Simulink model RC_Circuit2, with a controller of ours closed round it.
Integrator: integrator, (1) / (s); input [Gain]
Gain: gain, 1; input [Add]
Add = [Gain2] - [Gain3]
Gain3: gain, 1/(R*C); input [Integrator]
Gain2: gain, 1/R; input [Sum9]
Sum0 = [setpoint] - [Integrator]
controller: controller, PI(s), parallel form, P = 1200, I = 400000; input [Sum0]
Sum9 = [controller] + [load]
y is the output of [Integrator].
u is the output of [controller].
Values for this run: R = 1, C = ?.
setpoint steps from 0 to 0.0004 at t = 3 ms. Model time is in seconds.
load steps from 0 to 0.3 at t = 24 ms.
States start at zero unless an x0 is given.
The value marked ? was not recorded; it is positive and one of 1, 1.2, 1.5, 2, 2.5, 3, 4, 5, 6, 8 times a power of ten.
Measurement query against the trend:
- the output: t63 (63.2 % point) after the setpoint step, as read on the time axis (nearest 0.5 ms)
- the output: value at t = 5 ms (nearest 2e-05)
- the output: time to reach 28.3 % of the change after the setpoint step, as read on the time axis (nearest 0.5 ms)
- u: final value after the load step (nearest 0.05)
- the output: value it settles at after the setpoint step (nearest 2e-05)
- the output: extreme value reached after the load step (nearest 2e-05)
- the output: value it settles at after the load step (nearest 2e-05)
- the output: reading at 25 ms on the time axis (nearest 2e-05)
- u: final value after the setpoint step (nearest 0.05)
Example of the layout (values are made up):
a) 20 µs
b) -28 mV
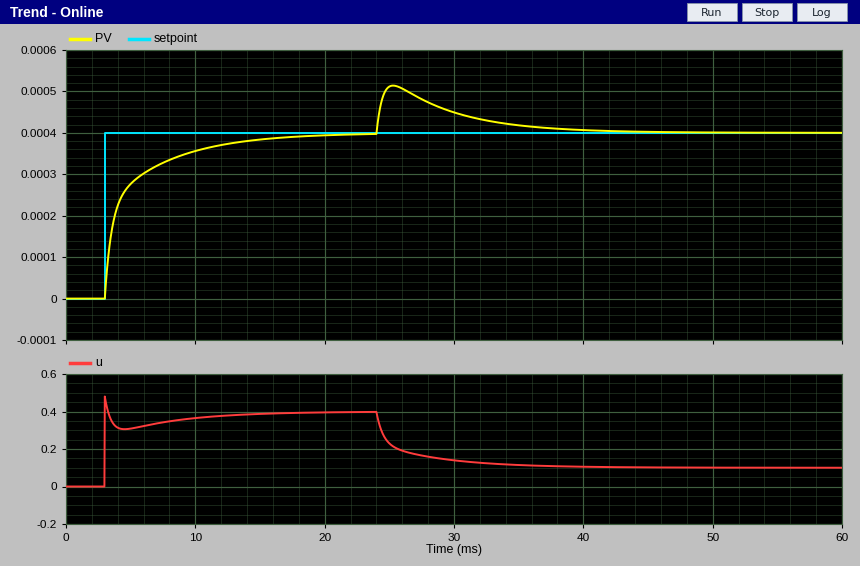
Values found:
a) 4.5 ms
b) 0.00028
c) 3.5 ms
d) 0.10
e) 0.00040
f) 0.00052
g) 0.00040
h) 0.00052
i) 0.40
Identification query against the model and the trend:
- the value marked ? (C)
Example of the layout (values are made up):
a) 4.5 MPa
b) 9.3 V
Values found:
a) 0.001
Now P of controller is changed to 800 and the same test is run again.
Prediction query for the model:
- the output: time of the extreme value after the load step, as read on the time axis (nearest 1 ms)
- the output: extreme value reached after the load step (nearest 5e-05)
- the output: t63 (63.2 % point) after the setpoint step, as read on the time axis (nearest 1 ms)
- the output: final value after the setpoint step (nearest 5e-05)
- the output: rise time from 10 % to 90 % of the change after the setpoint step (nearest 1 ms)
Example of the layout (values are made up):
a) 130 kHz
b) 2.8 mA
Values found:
a) 25 ms
b) 0.00055
c) 5 ms
d) 0.00040
e) 7 ms
